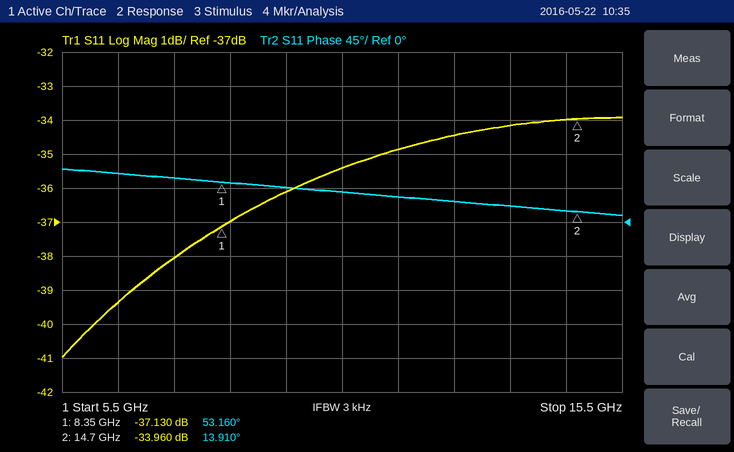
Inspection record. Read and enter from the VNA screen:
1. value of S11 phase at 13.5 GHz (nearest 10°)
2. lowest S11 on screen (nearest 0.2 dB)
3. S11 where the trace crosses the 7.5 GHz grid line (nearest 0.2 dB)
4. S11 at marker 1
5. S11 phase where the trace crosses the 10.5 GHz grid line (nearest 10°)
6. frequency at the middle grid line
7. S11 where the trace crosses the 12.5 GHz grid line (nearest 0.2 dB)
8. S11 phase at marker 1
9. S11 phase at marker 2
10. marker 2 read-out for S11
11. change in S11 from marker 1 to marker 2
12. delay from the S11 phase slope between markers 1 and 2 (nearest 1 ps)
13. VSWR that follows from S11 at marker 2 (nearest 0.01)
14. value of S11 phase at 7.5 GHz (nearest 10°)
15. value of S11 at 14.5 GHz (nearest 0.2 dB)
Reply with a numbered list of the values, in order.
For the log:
1. 20°
2. -41.0 dB
3. -38.0 dB
4. -37.130 dB
5. 40°
6. 10.5 GHz
7. -34.4 dB
8. 53.160°
9. 13.910°
10. -33.960 dB
11. 3.170 dB
12. 17 ps
13. 1.04
14. 60°
15. -34.0 dB
